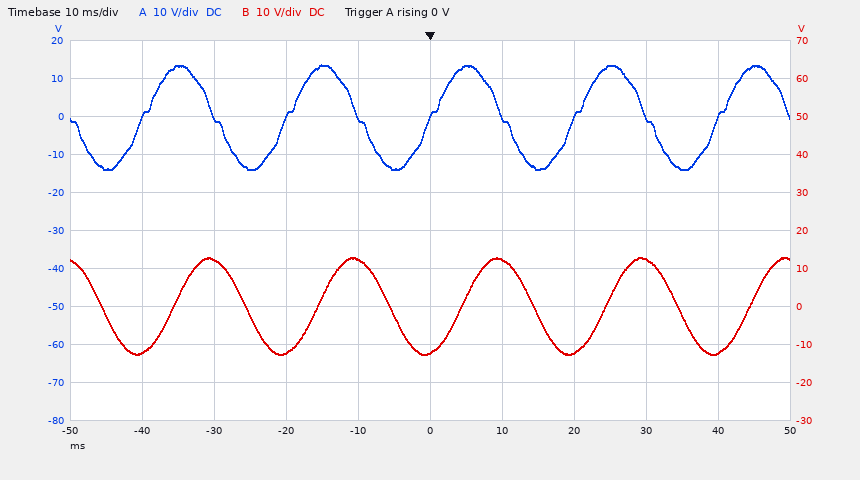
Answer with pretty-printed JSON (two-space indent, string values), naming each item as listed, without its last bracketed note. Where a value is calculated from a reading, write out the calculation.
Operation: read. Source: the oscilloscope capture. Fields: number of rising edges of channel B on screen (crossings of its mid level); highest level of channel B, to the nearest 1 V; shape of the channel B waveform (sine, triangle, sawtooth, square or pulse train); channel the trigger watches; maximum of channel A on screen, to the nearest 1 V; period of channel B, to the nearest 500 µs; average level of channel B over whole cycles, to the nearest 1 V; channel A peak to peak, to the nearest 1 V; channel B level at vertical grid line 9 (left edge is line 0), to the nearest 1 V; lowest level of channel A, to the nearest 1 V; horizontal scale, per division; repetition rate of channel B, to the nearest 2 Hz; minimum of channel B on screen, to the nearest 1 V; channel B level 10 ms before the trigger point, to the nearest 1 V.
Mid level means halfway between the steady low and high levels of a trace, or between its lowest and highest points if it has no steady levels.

{
  "number of rising edges of channel B on screen": "5",
  "highest level of channel B, to the nearest 1 V": "13 V",
  "shape of the channel B waveform": "sine",
  "channel the trigger watches": "channel A",
  "maximum of channel A on screen, to the nearest 1 V": "14 V",
  "period of channel B, to the nearest 500 µs": "20.0 ms",
  "average level of channel B over whole cycles, to the nearest 1 V": "(13 V + (-13 V)) / 2 ≈ 0 V",
  "channel A peak to peak, to the nearest 1 V": "14 V − (-14 V) = 28 V",
  "channel B level at vertical grid line 9 (left edge is line 0), to the nearest 1 V": "-12 V",
  "lowest level of channel A, to the nearest 1 V": "-14 V",
  "horizontal scale, per division": "10 ms",
  "repetition rate of channel B, to the nearest 2 Hz": "1 / 20.0 ms ≈ 50 Hz",
  "minimum of channel B on screen, to the nearest 1 V": "-13 V",
  "channel B level 10 ms before the trigger point, to the nearest 1 V": "12 V"
}
